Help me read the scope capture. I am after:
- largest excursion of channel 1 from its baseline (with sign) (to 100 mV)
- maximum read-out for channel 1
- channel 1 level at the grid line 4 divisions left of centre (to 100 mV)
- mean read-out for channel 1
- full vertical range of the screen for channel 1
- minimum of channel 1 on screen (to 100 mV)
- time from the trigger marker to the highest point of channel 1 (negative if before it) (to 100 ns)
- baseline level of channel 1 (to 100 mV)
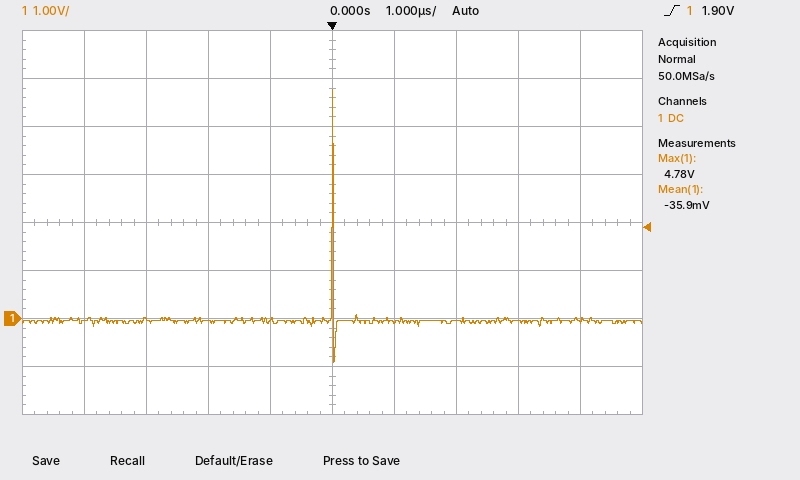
+4.8 V
4.78 V
-100 mV
-35.9 mV
8 V
-900 mV
0.0 µs
0.0 V
